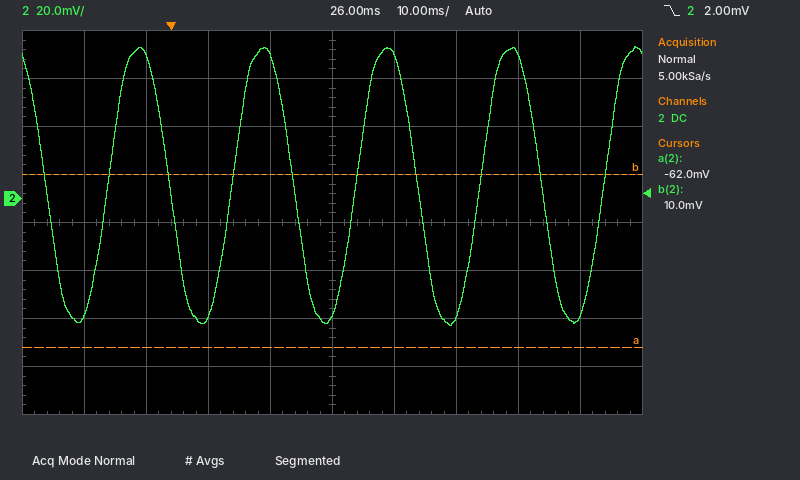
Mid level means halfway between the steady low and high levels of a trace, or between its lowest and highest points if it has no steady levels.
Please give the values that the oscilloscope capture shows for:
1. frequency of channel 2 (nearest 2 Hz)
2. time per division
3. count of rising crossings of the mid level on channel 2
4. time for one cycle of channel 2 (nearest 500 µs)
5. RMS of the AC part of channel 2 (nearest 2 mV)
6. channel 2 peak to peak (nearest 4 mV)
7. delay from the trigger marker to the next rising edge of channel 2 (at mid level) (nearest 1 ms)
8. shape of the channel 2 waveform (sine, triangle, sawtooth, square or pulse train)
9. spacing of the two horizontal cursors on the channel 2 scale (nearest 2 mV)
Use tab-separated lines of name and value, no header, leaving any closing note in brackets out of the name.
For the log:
frequency of channel 2	50 Hz
time per division	10 ms
count of rising crossings of the mid level on channel 2	5
time for one cycle of channel 2	20.0 ms
RMS of the AC part of channel 2	42 mV
channel 2 peak to peak	116 mV
delay from the trigger marker to the next rising edge of channel 2 (at mid level)	10 ms
shape of the channel 2 waveform	sine
spacing of the two horizontal cursors on the channel 2 scale	72 mV
